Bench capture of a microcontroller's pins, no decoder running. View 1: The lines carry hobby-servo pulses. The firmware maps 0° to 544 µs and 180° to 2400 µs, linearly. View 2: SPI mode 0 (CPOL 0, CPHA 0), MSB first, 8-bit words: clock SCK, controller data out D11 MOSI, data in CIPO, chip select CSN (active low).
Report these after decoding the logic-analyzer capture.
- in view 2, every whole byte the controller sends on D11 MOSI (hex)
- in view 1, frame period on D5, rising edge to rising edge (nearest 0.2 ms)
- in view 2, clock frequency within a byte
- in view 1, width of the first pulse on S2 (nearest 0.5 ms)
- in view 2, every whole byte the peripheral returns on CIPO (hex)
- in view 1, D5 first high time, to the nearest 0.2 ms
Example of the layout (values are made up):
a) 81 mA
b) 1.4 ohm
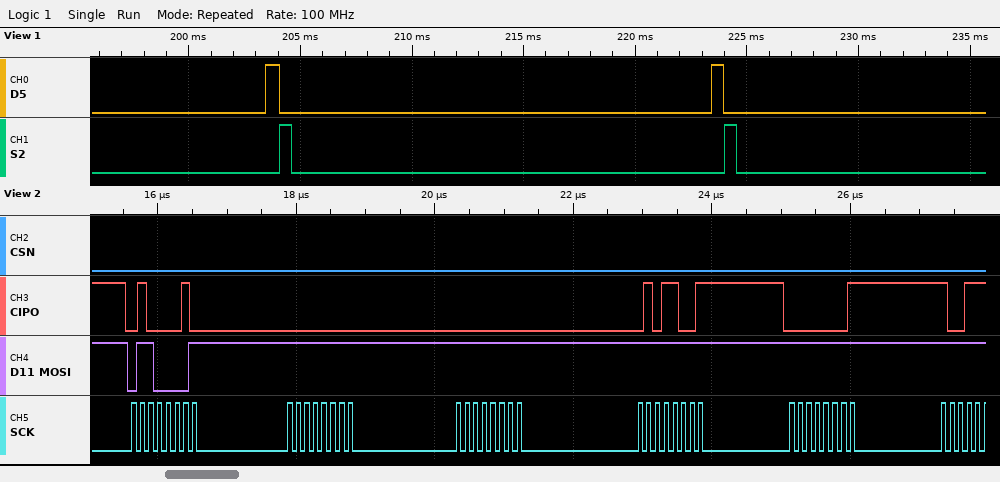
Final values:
a) 0x61 0xFF 0xFF 0xFF 0xFF
b) 20.0 ms
c) 8 MHz
d) 0.5 ms
e) 0x42 0x00 0x00 0x59 0x01
f) 0.6 ms
